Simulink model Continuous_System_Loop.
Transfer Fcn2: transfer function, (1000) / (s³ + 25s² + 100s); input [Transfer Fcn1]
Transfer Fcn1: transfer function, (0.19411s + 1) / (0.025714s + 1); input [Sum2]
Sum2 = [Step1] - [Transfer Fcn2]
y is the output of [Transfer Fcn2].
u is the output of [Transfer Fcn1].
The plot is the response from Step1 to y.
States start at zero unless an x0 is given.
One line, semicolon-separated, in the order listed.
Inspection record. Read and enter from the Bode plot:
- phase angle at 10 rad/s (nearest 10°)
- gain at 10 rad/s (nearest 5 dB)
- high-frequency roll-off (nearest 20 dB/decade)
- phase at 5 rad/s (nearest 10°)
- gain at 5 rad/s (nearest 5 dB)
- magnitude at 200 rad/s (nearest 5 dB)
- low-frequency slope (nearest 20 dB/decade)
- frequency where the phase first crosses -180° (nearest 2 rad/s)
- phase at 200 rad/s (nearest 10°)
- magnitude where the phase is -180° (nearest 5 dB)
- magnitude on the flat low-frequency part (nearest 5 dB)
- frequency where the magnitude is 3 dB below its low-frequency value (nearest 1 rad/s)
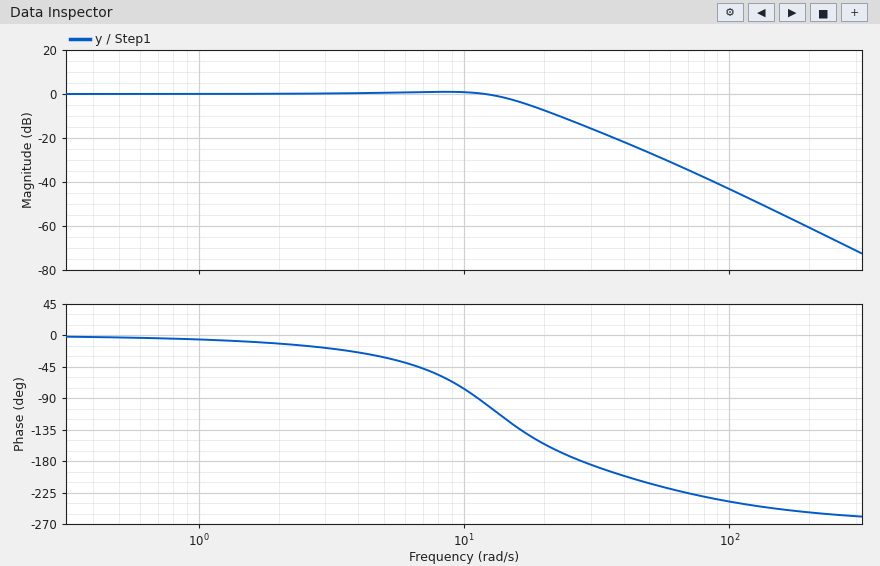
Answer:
-80°; 0 dB; -60 dB/decade; -30°; 0 dB; -60 dB; 0 dB/decade; 28 rad/s; -250°; -15 dB; 0 dB; 16 rad/s
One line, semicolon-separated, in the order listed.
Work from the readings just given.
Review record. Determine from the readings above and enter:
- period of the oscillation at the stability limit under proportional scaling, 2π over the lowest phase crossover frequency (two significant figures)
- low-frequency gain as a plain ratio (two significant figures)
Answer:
0.22 s; 1.0
